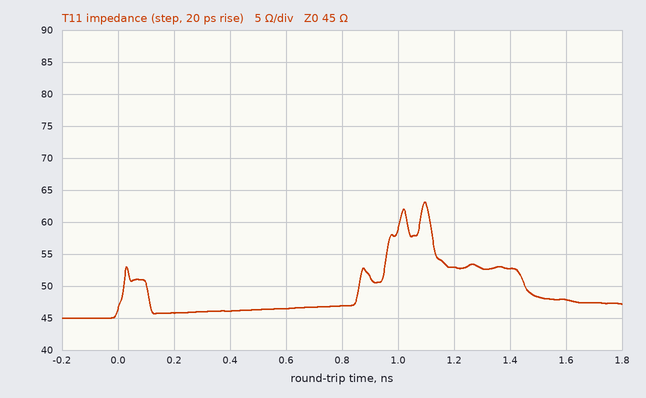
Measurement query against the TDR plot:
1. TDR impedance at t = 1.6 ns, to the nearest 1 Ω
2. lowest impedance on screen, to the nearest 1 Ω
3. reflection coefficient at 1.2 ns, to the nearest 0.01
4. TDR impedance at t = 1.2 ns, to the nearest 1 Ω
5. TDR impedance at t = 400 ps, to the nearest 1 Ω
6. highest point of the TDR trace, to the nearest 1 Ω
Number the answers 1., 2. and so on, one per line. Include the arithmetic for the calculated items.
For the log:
1. 48 Ω
2. 45 Ω
3. (53 − 45)/(53 + 45) ≈ +0.08
4. 53 Ω
5. 46 Ω
6. 63 Ω
